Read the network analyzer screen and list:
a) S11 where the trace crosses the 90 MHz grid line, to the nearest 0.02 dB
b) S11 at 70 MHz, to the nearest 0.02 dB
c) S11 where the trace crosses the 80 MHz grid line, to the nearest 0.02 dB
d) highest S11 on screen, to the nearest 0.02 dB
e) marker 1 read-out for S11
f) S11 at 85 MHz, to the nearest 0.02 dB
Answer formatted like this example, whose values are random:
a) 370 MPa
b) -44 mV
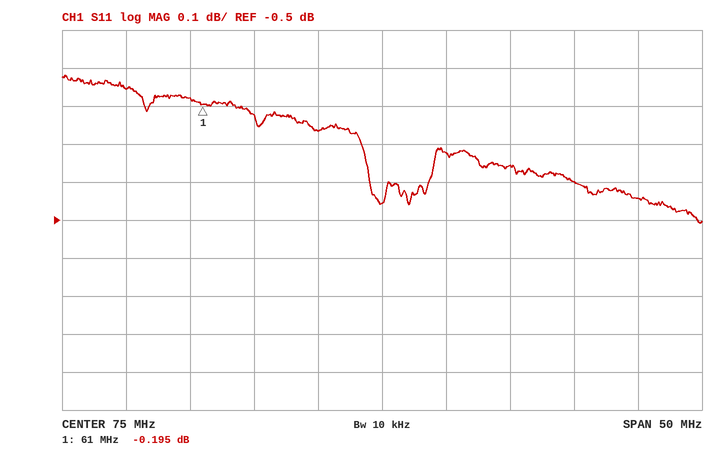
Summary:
a) -0.40 dB
b) -0.26 dB
c) -0.32 dB
d) -0.12 dB
e) -0.195 dB
f) -0.36 dB
